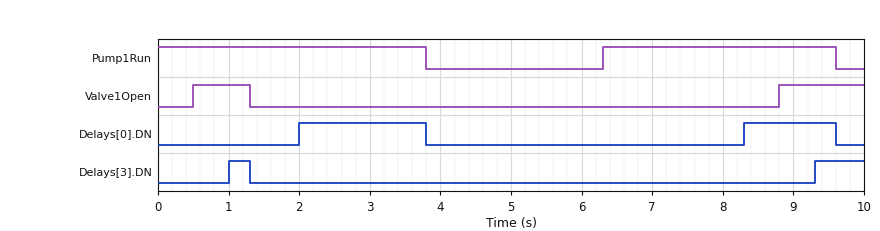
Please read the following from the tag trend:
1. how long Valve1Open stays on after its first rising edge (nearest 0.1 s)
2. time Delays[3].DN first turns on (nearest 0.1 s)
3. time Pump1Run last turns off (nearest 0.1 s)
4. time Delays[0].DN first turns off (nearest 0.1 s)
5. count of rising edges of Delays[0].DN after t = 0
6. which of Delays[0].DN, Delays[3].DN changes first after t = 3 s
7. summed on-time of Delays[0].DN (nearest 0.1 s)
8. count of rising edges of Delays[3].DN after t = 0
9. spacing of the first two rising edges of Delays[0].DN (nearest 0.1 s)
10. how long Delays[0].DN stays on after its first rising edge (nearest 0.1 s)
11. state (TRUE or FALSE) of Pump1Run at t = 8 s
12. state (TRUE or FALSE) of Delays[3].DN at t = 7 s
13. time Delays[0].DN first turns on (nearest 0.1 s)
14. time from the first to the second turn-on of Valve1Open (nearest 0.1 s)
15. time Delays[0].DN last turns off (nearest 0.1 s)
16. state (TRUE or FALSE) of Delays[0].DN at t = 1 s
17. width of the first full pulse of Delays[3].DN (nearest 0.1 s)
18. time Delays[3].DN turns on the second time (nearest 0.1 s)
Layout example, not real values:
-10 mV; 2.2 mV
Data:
0.8 s; 1.0 s; 9.6 s; 3.8 s; 2; Delays[0].DN; 3.1 s; 2; 6.3 s; 1.8 s; TRUE; FALSE; 2.0 s; 8.3 s; 9.6 s; FALSE; 0.3 s; 9.3 s
